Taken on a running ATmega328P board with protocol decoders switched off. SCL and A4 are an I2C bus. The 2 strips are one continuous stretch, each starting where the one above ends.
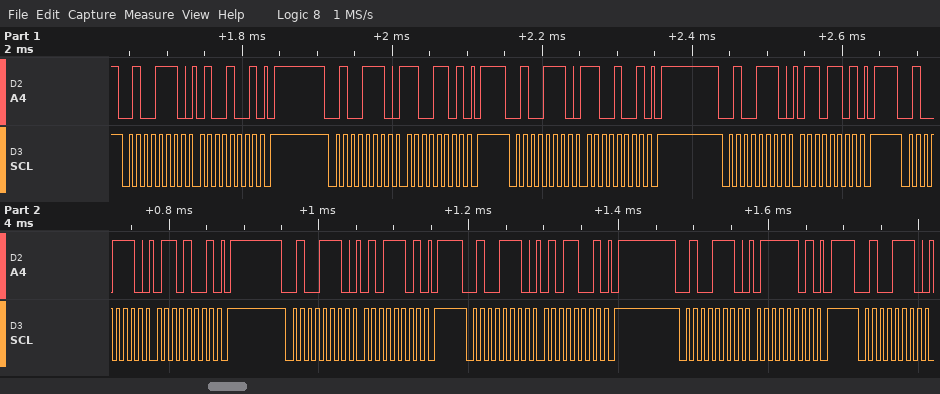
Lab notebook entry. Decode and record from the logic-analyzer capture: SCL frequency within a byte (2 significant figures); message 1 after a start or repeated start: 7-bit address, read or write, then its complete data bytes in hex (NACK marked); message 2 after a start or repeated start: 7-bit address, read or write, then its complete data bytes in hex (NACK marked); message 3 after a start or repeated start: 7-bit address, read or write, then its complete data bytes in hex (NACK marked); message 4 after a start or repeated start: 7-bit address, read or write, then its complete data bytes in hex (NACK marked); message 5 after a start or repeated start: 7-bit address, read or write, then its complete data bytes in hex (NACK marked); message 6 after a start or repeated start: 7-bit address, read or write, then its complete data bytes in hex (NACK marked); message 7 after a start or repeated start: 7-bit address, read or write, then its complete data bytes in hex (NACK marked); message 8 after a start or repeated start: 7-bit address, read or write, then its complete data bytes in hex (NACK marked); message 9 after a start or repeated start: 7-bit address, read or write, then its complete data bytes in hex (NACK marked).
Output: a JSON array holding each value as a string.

["100 kHz", "0x27 write: 49", "0x27 write: CD", "0x27 write: C9", "0x27 write: 6D", "0x27 write: 69", "0x27 write: 5D", "0x27 write: 59", "0x27 write: 7D", "0x27 write"]
